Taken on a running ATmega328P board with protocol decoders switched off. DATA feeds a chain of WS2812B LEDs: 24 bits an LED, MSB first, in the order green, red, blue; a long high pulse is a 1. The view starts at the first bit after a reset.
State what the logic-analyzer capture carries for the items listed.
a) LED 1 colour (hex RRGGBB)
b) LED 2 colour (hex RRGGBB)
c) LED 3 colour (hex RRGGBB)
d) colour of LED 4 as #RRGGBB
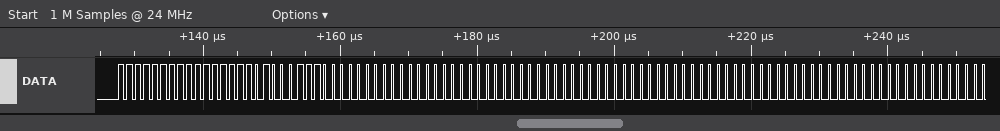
#FFFF47
#000000
#000000
#000000
